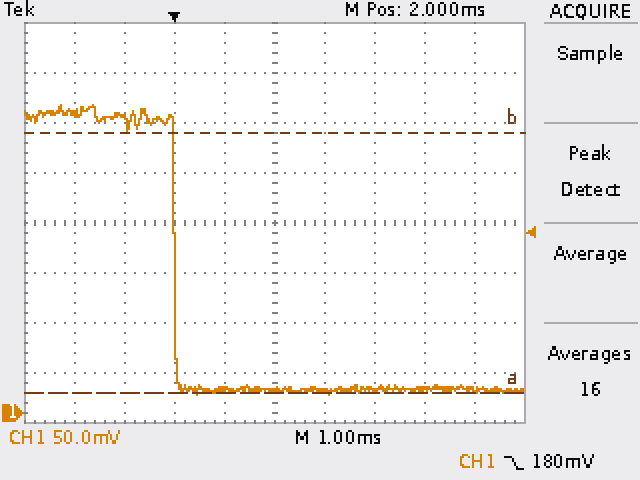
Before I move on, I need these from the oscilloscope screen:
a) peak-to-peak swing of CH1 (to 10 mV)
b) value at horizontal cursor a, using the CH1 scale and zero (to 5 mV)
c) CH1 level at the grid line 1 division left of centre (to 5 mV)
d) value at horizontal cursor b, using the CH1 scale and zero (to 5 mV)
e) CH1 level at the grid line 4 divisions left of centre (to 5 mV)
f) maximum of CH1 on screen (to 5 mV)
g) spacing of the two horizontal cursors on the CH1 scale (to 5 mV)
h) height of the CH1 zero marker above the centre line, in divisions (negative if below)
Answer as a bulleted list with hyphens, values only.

- 290 mV
- 20 mV
- 25 mV
- 280 mV
- 300 mV
- 310 mV
- 260 mV
- -3.8 div
